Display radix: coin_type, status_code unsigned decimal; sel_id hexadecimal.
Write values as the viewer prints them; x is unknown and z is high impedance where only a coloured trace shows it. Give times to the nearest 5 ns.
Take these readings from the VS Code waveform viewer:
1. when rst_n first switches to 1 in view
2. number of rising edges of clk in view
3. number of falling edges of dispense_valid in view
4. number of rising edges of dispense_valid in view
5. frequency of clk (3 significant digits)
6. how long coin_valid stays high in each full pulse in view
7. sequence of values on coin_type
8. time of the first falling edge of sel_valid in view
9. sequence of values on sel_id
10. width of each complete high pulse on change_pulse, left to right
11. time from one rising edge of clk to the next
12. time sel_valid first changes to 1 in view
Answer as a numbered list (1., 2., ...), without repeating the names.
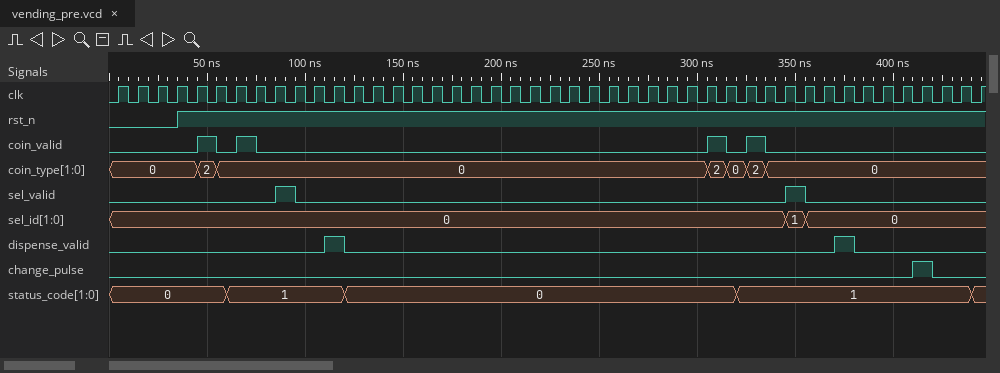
1. 35 ns
2. 45
3. 2
4. 2
5. 100 MHz
6. 10 ns, 10 ns, 10 ns, 10 ns
7. 0, 2, 0, 2, 0, 2, 0
8. 95 ns
9. 0, 1, 0
10. 10 ns
11. 10 ns
12. 85 ns
